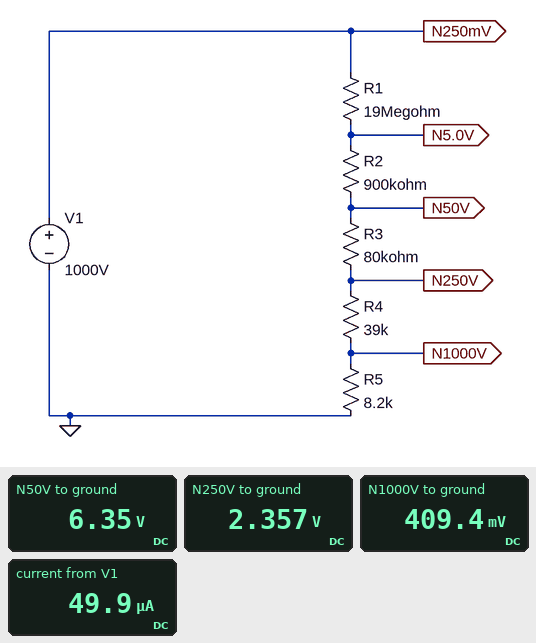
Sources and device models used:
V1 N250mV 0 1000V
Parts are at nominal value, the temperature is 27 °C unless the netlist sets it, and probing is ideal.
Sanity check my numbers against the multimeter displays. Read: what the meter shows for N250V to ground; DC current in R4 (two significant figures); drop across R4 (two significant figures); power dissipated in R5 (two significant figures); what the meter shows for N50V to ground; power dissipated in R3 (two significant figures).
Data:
2.357 V
50 µA
1.9 V
20 µW
6.35 V
200 µW
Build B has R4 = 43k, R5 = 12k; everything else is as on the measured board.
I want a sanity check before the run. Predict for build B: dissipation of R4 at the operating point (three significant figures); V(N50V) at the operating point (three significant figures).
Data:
107 µW
6.74 V
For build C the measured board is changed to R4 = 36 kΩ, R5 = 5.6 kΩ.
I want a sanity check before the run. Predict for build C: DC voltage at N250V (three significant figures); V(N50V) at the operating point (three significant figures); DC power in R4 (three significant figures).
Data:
2.08 V
6.07 V
89.8 µW
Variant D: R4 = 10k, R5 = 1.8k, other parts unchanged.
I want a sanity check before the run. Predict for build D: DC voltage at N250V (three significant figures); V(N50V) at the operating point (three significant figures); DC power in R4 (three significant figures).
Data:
590 mV
4.59 V
25.0 µW
